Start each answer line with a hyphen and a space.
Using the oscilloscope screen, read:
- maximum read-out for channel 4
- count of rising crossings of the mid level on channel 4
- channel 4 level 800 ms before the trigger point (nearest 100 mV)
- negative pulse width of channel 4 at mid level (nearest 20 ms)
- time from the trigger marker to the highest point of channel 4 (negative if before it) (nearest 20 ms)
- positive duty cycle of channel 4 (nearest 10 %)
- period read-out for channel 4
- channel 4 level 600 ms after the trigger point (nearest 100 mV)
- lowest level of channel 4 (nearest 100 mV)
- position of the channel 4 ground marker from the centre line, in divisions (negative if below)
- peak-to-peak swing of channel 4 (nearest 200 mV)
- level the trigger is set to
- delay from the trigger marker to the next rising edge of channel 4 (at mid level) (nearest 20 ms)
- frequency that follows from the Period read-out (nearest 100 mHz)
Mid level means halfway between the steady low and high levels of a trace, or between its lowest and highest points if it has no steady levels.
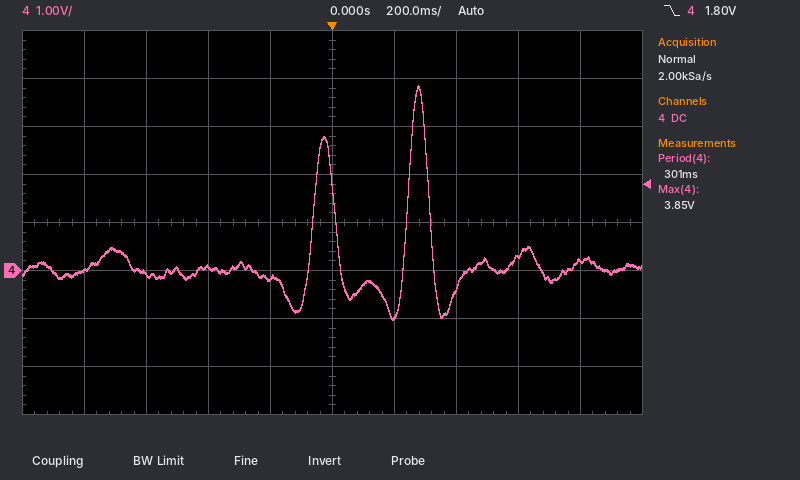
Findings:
- 3.85 V
- 2
- 0.0 V
- 240 ms
- +280 ms
- 20 %
- 301 ms
- 300 mV
- -1.0 V
- -1.0 div
- 4.8 V
- 1.80 V
- 240 ms
- 3.3 Hz
